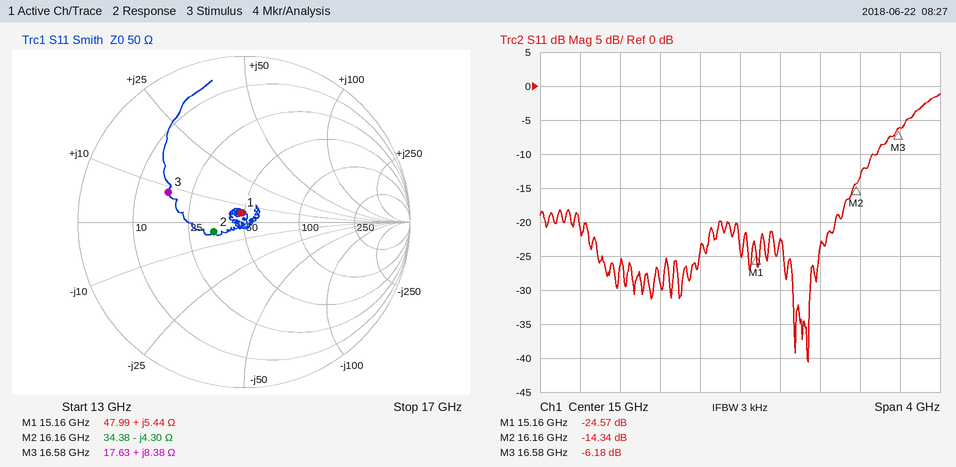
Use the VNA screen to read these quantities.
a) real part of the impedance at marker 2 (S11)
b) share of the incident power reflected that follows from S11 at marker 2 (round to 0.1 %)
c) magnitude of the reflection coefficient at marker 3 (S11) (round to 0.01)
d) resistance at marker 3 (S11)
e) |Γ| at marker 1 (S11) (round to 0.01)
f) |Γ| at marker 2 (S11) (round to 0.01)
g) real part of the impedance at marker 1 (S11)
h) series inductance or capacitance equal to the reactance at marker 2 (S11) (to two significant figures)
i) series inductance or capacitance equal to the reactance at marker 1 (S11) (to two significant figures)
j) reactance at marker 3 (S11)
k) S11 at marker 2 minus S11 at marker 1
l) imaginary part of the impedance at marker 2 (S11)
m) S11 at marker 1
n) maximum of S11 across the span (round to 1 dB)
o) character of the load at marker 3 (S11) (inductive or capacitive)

34.38 Ω
3.7 %
0.49
17.63 Ω
0.06
0.19
47.99 Ω
2.3 pF
57 pH
+8.38 Ω
10.23 dB
-4.30 Ω
-24.57 dB
-1 dB
inductive
